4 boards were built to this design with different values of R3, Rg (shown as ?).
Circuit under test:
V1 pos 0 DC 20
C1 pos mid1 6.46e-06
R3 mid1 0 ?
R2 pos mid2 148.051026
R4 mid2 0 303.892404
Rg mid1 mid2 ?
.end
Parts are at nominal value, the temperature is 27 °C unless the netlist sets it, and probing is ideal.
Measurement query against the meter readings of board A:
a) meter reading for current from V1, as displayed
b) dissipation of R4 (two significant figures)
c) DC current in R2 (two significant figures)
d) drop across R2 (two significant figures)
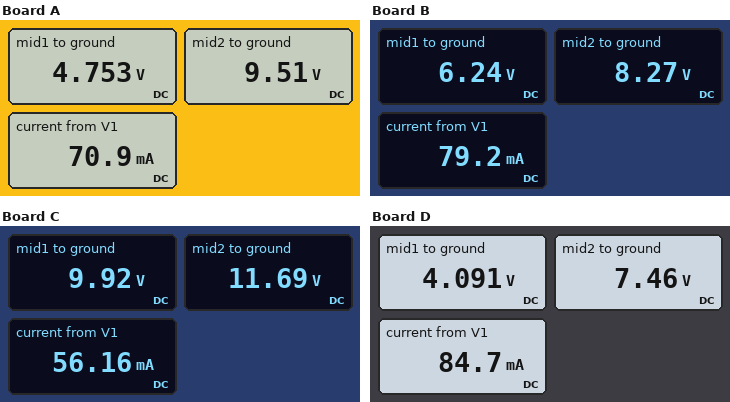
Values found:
70.9 mA
300 mW
71 mA
10 V
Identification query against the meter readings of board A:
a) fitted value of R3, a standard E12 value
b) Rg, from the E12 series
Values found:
120 Ω
120 Ω
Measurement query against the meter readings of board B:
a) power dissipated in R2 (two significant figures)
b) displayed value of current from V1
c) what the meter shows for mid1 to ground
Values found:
930 mW
79.2 mA
6.24 V
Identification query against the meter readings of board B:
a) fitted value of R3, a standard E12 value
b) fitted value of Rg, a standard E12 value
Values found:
120 Ω
39 Ω
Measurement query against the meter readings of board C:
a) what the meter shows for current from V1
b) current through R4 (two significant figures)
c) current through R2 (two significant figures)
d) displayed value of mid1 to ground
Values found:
56.16 mA
38 mA
56 mA
9.92 V
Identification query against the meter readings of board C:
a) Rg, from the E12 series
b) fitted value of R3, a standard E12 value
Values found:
100 Ω
560 Ω
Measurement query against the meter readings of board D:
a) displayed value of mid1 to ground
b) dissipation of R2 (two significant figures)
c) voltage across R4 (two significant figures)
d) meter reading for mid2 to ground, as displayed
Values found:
4.091 V
1.1 W
7.5 V
7.46 V
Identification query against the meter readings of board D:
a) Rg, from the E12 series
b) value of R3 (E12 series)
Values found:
56 Ω
68 Ω
